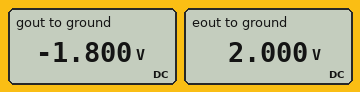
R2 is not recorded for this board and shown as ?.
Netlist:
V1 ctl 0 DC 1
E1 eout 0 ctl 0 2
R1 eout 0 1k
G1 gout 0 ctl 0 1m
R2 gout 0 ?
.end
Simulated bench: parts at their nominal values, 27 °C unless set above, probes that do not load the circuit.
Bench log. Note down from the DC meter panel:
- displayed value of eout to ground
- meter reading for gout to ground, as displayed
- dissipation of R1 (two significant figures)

2.000 V
-1.800 V
4.0 mW
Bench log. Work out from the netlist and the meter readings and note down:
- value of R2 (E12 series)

1.8 kΩ
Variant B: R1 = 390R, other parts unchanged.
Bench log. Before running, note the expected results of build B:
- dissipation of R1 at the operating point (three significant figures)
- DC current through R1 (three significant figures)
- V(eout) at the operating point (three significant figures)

10.3 mW
5.13 mA
2.00 V
